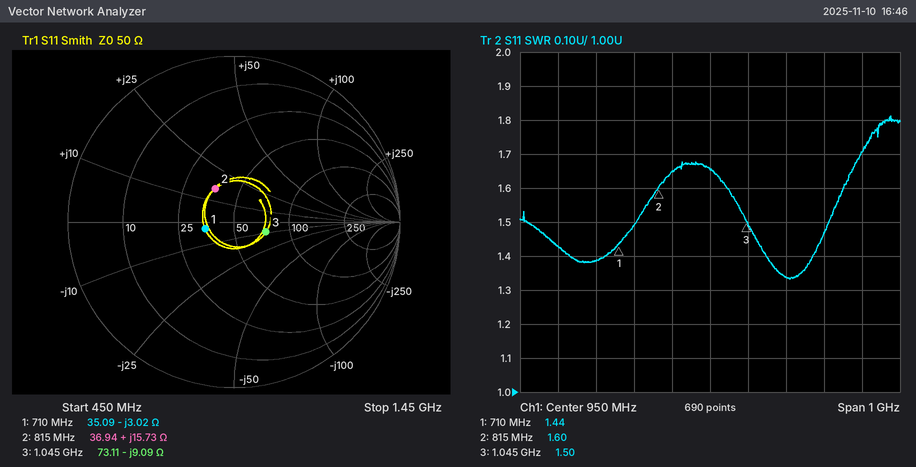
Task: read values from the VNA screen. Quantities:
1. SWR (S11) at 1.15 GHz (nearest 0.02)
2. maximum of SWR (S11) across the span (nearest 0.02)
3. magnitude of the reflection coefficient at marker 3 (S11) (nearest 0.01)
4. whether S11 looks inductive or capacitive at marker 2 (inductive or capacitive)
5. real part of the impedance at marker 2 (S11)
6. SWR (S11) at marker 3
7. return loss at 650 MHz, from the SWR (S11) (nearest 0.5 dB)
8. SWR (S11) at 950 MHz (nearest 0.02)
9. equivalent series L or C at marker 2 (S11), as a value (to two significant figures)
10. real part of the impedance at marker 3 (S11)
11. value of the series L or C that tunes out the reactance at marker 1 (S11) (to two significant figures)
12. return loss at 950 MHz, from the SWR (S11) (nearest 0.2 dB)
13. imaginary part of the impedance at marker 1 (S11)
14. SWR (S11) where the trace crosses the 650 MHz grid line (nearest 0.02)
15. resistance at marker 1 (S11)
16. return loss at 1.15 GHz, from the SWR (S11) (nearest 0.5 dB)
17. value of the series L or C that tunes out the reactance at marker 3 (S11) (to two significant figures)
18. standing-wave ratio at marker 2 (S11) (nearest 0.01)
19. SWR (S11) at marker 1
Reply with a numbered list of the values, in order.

1. 1.34
2. 1.82
3. 0.20
4. inductive
5. 36.94 Ω
6. 1.50
7. 16.0 dB
8. 1.66
9. 3.1 nH
10. 73.11 Ω
11. 680 pH
12. 12.2 dB
13. -3.02 Ω
14. 1.38
15. 35.09 Ω
16. 17.0 dB
17. 1.4 nH
18. 1.60
19. 1.44
